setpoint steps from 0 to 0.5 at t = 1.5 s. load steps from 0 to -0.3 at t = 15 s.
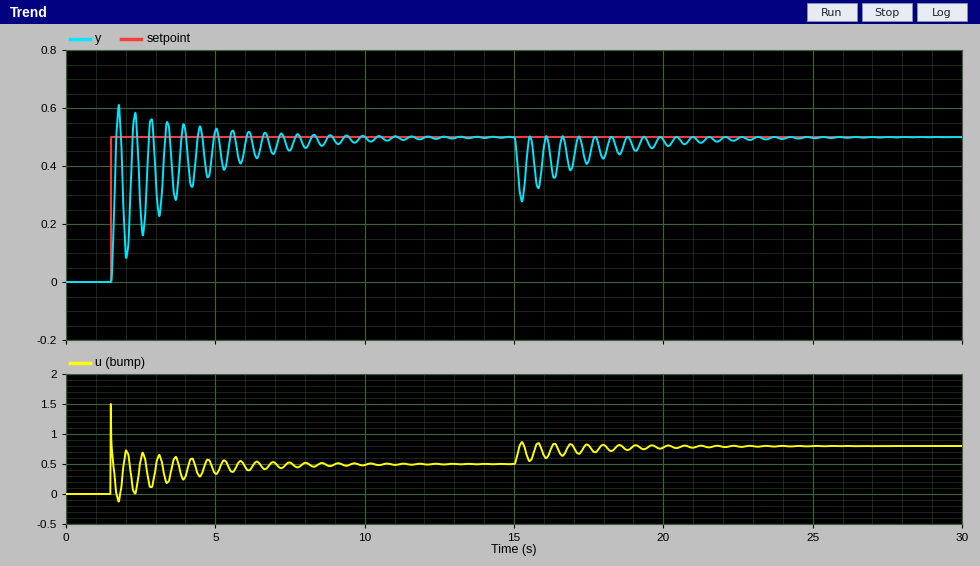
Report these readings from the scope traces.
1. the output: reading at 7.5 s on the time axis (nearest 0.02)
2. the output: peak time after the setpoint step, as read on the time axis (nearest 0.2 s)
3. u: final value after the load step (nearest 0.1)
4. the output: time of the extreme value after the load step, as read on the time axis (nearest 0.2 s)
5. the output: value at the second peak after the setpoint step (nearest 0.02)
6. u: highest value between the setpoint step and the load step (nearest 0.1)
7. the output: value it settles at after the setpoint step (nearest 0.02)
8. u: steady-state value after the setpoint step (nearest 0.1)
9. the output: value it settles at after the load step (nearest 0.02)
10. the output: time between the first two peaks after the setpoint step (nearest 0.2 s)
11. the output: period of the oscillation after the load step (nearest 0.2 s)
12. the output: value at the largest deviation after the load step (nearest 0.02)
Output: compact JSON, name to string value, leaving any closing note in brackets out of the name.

{"the output: reading at 7.5 s on the time axis": "0.46", "the output: peak time after the setpoint step, as read on the time axis": "1.8 s", "u: final value after the load step": "0.8", "the output: time of the extreme value after the load step, as read on the time axis": "15.2 s", "the output: value at the second peak after the setpoint step": "0.58", "u: highest value between the setpoint step and the load step": "1.5", "the output: value it settles at after the setpoint step": "0.50", "u: steady-state value after the setpoint step": "0.5", "the output: value it settles at after the load step": "0.50", "the output: time between the first two peaks after the setpoint step": "0.6 s", "the output: period of the oscillation after the load step": "0.6 s", "the output: value at the largest deviation after the load step": "0.28"}
